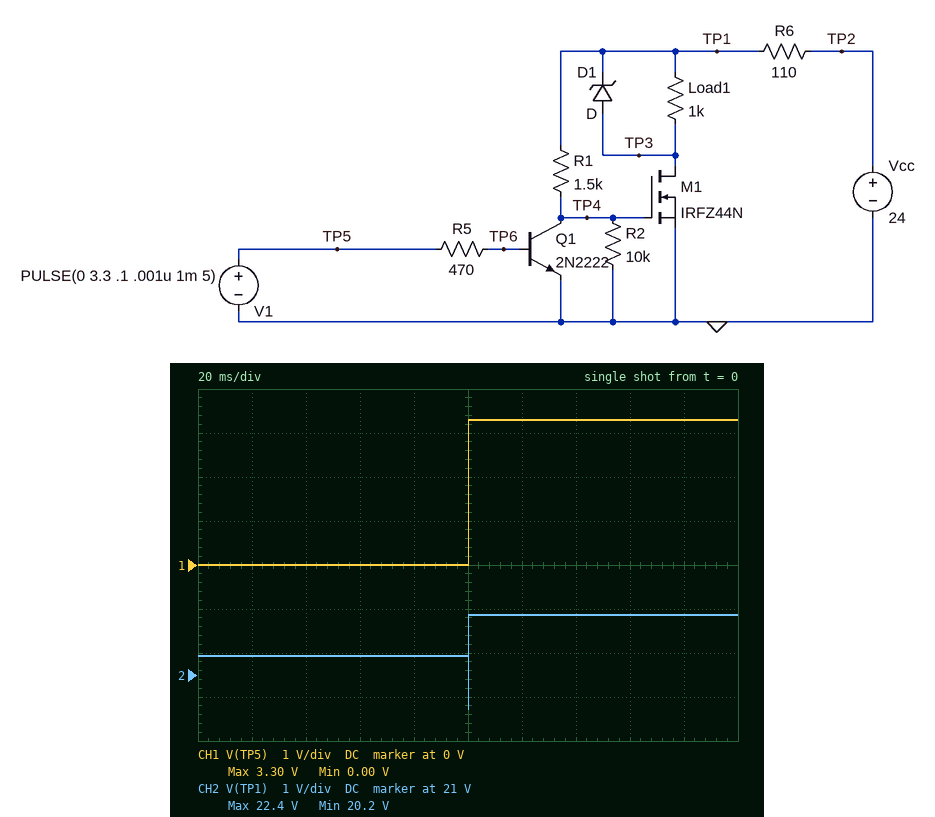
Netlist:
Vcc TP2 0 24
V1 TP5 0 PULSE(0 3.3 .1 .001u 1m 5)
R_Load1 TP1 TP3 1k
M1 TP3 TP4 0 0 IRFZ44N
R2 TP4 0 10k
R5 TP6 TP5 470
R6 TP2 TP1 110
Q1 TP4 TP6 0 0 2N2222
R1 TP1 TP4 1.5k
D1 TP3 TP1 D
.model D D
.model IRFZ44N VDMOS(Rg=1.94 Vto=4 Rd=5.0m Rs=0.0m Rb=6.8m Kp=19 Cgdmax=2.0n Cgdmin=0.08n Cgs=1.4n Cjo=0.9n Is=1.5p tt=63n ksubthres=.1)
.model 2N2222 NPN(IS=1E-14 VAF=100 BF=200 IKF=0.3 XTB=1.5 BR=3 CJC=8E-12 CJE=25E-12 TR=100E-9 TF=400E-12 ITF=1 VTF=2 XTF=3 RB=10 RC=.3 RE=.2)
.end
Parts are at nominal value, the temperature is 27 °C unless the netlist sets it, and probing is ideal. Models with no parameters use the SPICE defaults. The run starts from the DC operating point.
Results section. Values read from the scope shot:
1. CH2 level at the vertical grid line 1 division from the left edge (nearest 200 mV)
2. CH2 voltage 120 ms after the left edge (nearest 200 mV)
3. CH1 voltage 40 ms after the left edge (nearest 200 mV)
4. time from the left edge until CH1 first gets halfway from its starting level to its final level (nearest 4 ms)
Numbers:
21.4 V
22.4 V
0 V
100 ms
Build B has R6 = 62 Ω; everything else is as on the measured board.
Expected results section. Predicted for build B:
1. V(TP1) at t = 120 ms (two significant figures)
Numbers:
23 V
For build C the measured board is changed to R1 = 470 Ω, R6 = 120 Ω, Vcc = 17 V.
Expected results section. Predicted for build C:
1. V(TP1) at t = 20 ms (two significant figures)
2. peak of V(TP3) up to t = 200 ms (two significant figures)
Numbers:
15 V
14 V
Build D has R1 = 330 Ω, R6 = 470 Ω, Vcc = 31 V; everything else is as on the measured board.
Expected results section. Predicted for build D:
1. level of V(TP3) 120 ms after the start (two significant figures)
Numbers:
13 V
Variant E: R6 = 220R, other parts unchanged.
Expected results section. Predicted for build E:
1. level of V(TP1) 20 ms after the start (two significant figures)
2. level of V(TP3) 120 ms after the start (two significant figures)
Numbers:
19 V
21 V
